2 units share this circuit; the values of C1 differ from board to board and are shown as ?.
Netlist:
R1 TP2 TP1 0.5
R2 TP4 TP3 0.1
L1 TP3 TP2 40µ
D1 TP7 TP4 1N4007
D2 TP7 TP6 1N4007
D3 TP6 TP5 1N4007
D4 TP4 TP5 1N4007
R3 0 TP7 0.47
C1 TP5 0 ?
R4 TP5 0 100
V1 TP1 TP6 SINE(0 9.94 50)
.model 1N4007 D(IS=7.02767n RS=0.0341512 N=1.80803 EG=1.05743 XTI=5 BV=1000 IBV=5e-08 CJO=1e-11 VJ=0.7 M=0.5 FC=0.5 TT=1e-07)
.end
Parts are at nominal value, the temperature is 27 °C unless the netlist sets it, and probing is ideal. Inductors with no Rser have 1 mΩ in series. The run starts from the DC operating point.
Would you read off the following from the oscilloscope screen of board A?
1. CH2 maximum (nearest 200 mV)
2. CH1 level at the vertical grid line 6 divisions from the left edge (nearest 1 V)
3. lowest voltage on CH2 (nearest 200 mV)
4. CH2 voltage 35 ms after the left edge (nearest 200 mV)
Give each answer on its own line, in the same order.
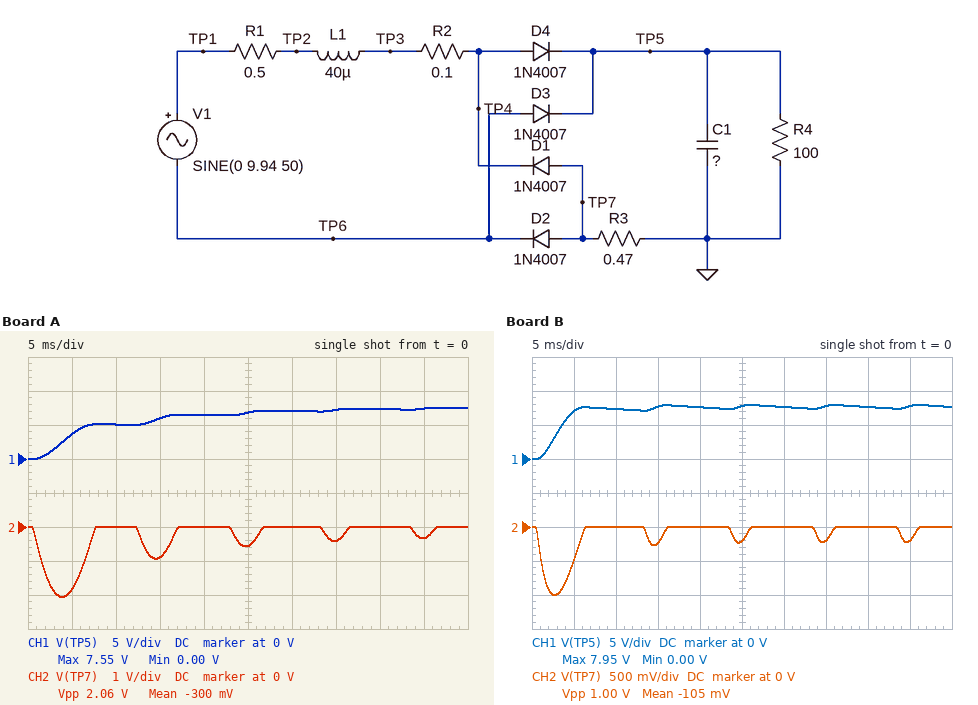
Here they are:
0 V
7 V
-2.0 V
-400 mV
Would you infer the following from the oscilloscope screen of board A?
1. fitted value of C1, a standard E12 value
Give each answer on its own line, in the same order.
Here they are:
3.9 mF
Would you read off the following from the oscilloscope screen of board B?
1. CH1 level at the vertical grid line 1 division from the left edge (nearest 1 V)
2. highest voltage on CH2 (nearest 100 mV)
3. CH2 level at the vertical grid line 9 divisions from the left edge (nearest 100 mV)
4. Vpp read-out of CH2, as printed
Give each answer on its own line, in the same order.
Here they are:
7 V
0 V
-200 mV
1.00 V
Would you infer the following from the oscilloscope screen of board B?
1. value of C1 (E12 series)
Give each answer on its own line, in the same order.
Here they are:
1 mF
